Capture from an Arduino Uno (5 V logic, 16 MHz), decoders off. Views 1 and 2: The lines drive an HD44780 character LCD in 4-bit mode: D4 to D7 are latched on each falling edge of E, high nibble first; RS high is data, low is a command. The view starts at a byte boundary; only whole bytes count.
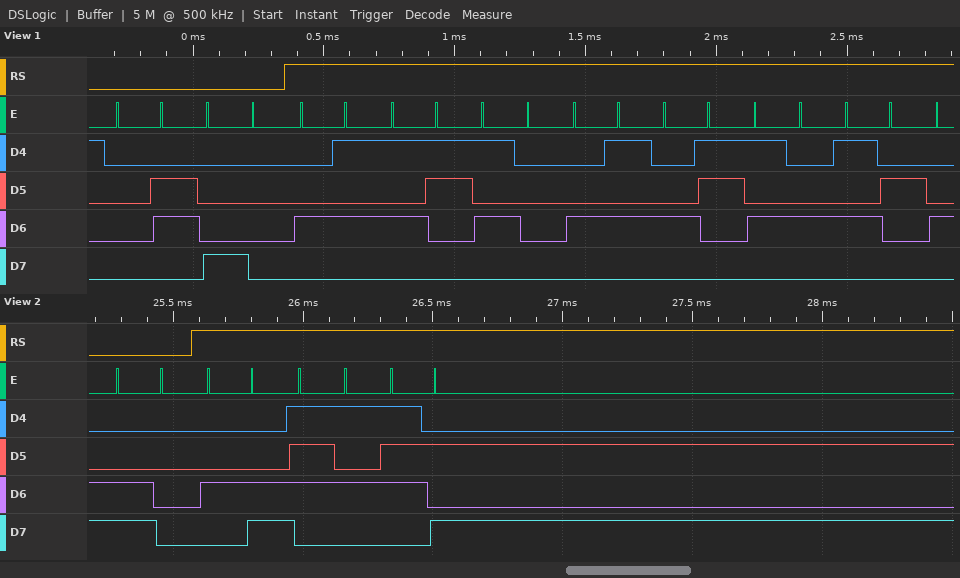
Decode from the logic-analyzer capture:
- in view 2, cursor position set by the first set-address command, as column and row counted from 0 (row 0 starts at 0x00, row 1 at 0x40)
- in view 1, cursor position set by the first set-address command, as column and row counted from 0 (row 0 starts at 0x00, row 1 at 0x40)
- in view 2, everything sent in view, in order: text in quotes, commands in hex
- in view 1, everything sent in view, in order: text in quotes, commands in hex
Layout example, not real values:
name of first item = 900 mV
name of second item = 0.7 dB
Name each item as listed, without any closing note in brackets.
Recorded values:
in view 2, cursor position set by the first set-address command, as column and row counted from 0 = column 0, row 1
in view 1, cursor position set by the first set-address command, as column and row counted from 0 = column 0, row 0
in view 2, everything sent in view, in order: text in quotes, commands in hex = 0xC0 "Luz"
in view 1, everything sent in view, in order: text in quotes, commands in hex = 0x06 0x80 "ESPECTR"
